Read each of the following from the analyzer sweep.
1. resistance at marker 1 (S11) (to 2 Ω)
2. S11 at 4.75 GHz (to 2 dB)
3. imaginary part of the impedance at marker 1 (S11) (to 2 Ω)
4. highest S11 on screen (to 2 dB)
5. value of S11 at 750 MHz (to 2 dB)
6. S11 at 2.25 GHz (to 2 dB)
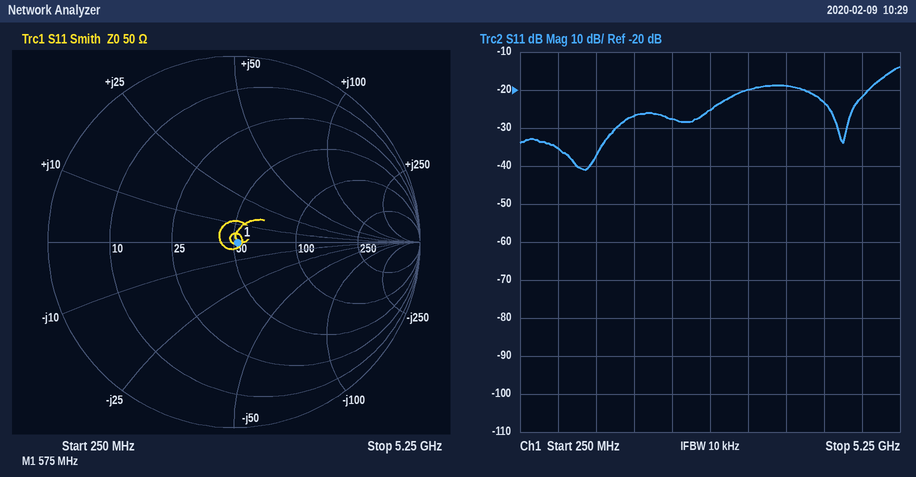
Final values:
52 Ω
-22 dB
0 Ω
-14 dB
-36 dB
-28 dB
